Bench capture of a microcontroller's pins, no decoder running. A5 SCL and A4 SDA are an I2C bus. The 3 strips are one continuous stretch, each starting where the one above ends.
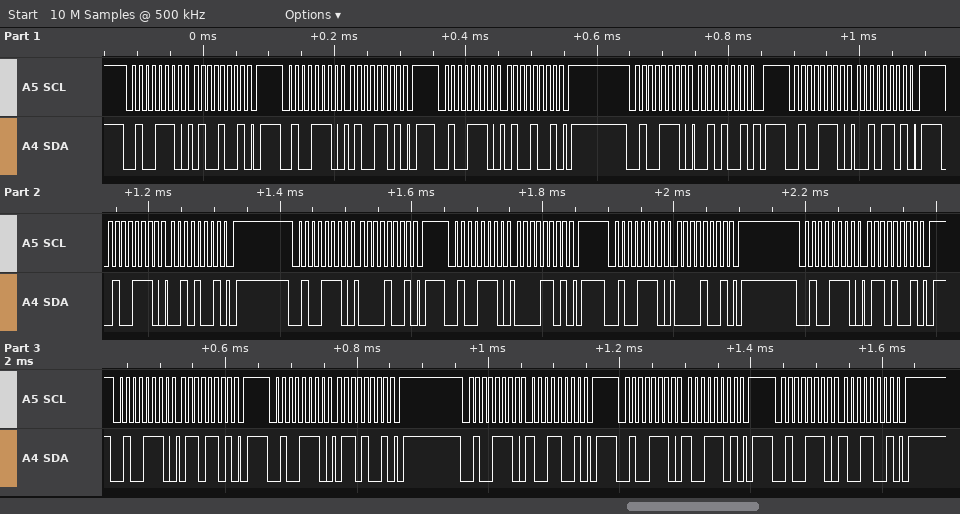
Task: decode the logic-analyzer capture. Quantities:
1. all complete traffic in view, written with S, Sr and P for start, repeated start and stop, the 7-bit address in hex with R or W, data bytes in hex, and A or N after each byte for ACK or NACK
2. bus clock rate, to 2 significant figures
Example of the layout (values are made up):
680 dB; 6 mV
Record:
S 27W A 49 A P S 27W A 4D A P S 27W A 49 A P S 27W A 29 A P S 27W A 2D A P S 27W A 29 A P S 27W A 09 A P S 27W A 0D A P S 27W A 09 A P S 27W A 69 A P S 27W A 6D A P S 27W A 69 A P S 27W A 99 A P S 27W A 9D A P S 27W A 99 A P; 100 kHz
